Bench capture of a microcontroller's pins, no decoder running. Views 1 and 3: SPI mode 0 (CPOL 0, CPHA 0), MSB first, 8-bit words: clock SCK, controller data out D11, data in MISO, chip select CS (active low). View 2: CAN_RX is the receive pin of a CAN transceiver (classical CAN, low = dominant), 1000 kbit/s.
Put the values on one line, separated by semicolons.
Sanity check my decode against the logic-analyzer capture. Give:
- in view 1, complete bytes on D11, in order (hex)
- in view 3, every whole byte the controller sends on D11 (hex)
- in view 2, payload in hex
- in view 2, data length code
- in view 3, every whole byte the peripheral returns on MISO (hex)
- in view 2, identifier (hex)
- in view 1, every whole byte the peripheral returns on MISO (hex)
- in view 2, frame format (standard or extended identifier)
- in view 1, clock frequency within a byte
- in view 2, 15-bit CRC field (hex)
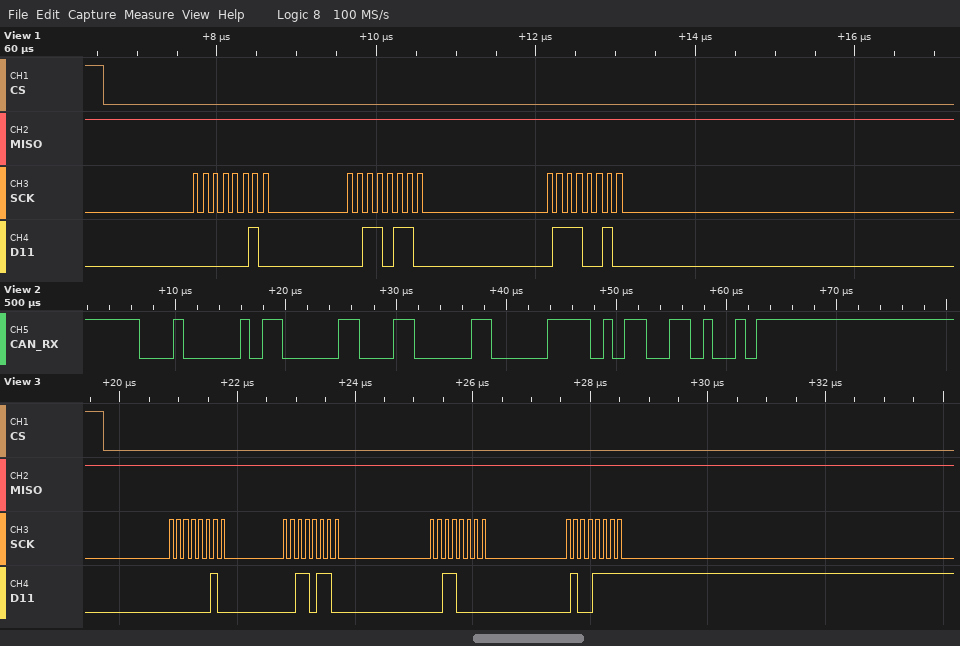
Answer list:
0x02 0x36 0x72; 02 36 30 4F; 30 41; 2; FF FF FF FF; 0x103; 0xFF 0xFF 0xFF; standard; 8 MHz; 0x6B34
